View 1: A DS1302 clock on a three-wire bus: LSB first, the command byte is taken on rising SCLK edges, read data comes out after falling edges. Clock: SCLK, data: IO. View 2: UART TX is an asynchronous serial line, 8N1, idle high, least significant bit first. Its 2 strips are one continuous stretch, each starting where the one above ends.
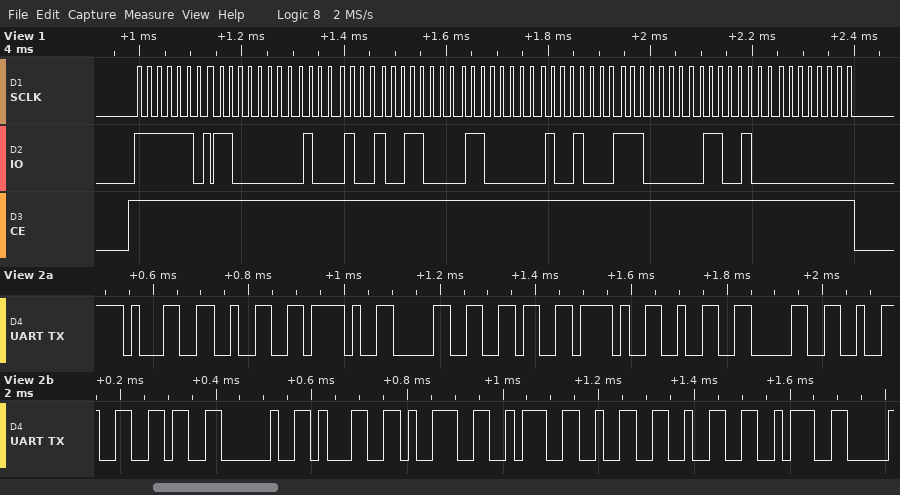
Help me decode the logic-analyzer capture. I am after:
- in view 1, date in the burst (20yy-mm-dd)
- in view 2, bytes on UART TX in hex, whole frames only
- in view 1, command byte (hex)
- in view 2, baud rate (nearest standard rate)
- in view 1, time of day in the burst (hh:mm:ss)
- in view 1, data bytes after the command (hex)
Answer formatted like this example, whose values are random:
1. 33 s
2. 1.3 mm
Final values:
1. 2026-12-06
2. 31 32 2F 30 36 2F 32 30 32 36 20 31 39 3A 32 32 3A
3. 0xBF
4. 57600 baud
5. 19:22:03
6. 03 22 19 06 12 07 26 00
